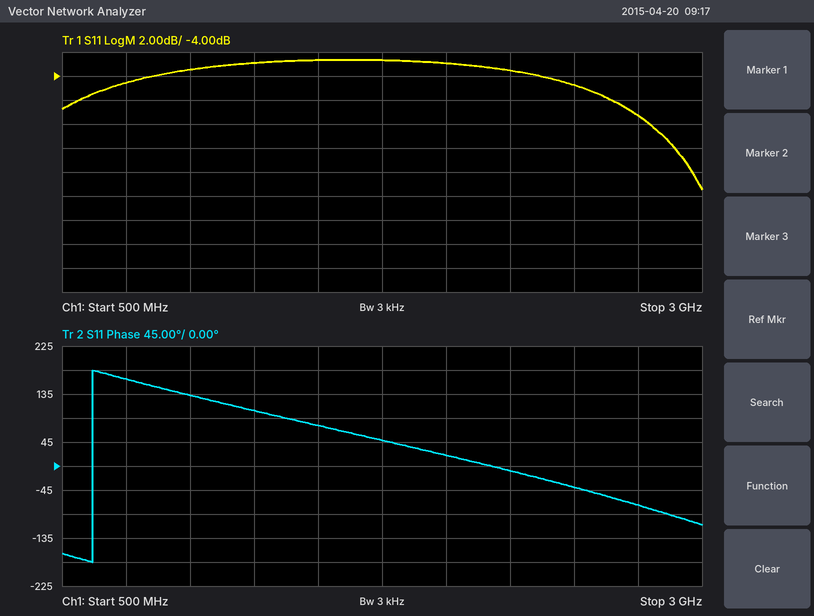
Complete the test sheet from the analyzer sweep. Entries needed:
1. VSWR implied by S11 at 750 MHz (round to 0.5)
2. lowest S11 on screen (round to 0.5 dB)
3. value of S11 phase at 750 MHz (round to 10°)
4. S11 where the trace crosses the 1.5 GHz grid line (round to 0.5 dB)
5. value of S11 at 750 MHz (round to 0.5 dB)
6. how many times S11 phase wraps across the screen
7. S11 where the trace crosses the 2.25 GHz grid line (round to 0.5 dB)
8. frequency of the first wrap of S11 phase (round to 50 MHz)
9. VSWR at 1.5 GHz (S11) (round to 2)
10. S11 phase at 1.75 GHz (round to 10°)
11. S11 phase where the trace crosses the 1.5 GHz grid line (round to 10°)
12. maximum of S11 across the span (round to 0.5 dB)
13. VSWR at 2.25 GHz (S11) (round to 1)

4.0
-13.5 dB
160°
-2.5 dB
-4.5 dB
1
-3.5 dB
600 MHz
6
50°
80°
-2.5 dB
5
